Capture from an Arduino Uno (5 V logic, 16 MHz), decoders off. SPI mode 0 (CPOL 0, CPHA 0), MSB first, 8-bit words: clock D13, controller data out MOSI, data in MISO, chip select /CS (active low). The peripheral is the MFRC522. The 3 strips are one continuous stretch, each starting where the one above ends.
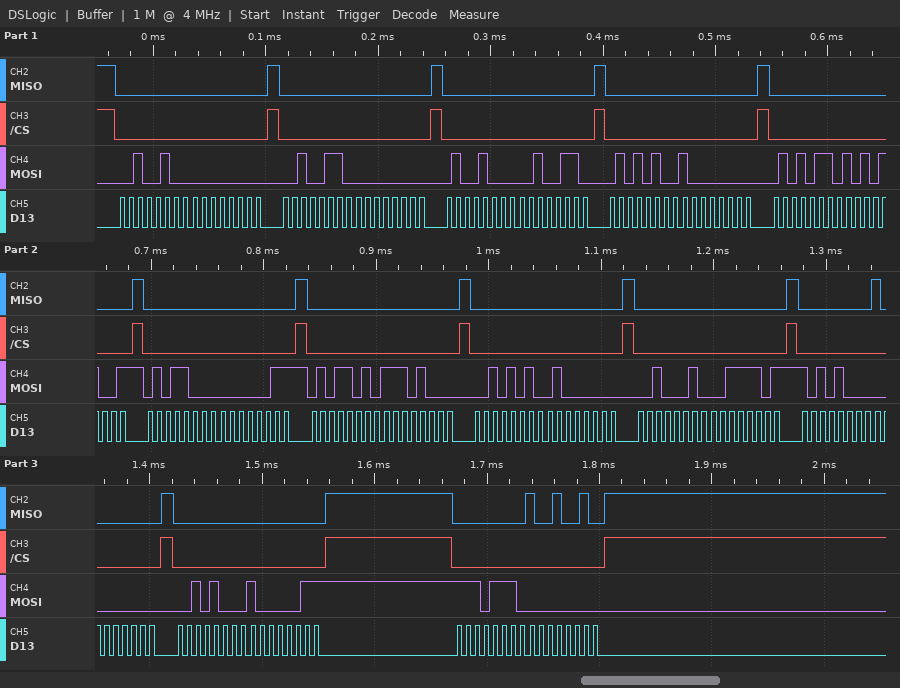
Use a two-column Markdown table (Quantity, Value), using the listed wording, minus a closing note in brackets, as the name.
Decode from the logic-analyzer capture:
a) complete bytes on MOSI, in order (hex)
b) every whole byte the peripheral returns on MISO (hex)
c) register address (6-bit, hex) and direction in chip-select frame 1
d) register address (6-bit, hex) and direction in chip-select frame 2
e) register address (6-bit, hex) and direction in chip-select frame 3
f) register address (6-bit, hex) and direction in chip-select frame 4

| Quantity | Value |
|---|---|
| complete bytes on MOSI, in order | 24 00 26 00 48 26 54 80 56 A9 58 03 5A E8 2A 40 22 3D A8 00 28 83 EE 00 |
| every whole byte the peripheral returns on MISO | 00 00 00 00 00 00 00 00 00 00 00 00 00 00 00 00 00 00 00 80 00 00 00 92 |
| register address (6-bit, hex) and direction in chip-select frame 1 | 0x12 write |
| register address (6-bit, hex) and direction in chip-select frame 2 | 0x13 write |
| register address (6-bit, hex) and direction in chip-select frame 3 | 0x24 write |
| register address (6-bit, hex) and direction in chip-select frame 4 | 0x2A write |
